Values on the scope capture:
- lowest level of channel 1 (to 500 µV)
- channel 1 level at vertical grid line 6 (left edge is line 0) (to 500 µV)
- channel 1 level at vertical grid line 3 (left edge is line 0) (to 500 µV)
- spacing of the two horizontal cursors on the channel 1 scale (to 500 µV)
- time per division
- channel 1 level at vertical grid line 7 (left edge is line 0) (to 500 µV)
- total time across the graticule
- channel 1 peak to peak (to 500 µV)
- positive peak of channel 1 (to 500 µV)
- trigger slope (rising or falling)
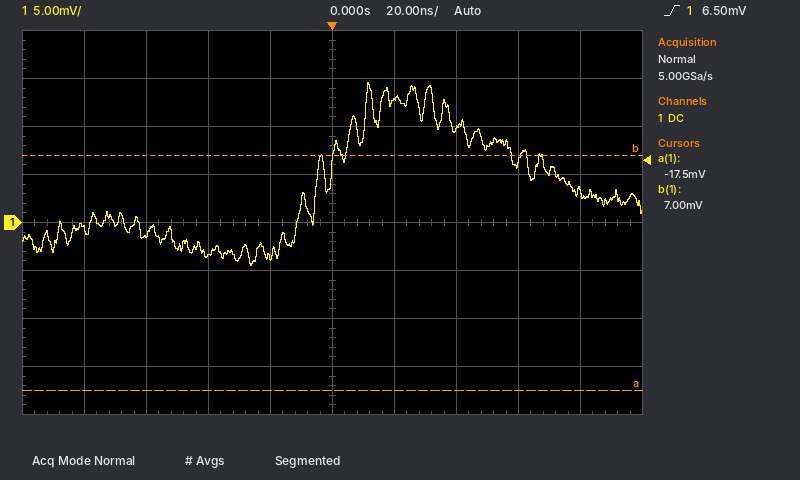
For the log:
-4.5 mV
13.0 mV
-3.5 mV
24.5 mV
20 ns
10.0 mV
200 ns
19.0 mV
14.5 mV
rising
